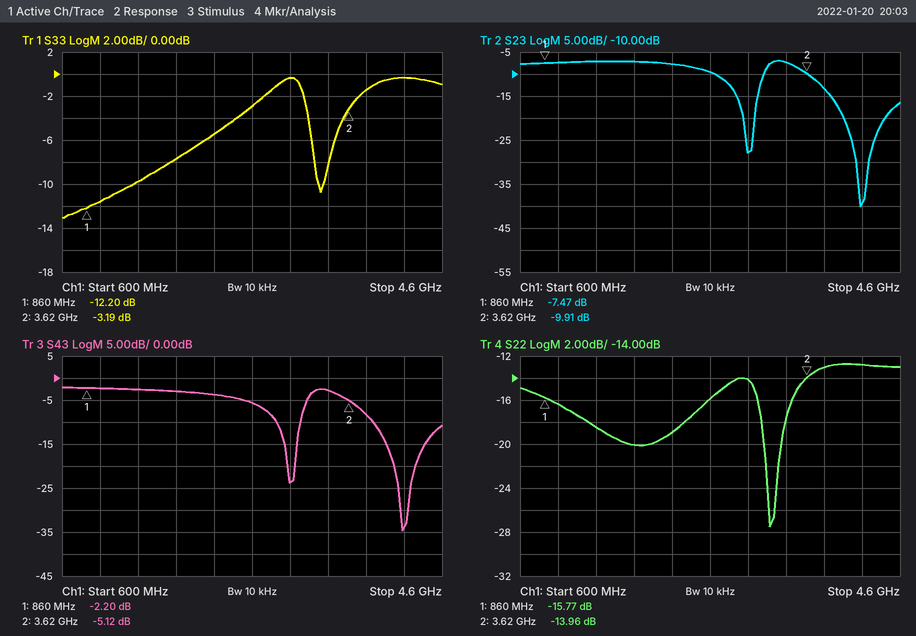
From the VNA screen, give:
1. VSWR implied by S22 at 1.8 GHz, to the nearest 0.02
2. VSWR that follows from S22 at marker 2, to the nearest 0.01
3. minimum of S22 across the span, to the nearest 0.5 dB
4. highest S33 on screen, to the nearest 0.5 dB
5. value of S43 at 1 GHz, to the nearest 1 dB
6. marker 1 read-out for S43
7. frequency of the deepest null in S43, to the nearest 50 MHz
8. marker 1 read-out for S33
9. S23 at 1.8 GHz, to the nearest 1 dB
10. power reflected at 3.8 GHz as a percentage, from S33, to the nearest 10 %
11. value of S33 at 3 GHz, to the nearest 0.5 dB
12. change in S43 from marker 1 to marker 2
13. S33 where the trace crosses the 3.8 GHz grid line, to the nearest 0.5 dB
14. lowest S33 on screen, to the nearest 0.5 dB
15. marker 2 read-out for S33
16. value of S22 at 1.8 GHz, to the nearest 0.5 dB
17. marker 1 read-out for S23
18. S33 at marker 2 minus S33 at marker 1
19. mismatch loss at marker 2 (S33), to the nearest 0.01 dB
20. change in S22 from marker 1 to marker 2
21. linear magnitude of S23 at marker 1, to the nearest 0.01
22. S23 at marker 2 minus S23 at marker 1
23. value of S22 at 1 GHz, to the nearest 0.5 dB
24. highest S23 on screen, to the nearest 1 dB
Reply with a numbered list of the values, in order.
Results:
1. 1.22
2. 1.50
3. -27.5 dB
4. -0.5 dB
5. -2 dB
6. -2.20 dB
7. 4.20 GHz
8. -12.20 dB
9. -7 dB
10. 70 %
11. -0.5 dB
12. -2.92 dB
13. -1.5 dB
14. -13.0 dB
15. -3.19 dB
16. -20.0 dB
17. -7.47 dB
18. 9.01 dB
19. 2.84 dB
20. 1.81 dB
21. 0.42
22. -2.44 dB
23. -16.5 dB
24. -7 dB
